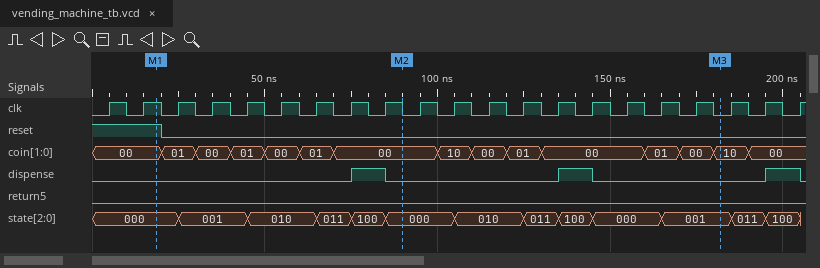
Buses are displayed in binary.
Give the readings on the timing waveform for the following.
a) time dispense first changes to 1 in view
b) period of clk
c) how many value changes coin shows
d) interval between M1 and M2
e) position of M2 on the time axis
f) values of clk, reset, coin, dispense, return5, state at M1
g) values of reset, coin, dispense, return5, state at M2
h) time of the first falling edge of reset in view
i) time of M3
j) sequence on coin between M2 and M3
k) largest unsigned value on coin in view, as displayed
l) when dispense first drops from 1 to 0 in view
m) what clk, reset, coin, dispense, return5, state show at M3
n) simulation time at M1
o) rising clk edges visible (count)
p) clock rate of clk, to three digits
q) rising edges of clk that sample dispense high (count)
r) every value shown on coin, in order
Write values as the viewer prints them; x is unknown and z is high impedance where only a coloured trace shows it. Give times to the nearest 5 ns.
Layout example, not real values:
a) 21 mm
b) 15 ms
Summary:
a) 75 ns
b) 10 ns
c) 14
d) 70 ns
e) 90 ns
f) clk=1, reset=1, coin=00, dispense=0, return5=0, state=000
g) reset=0, coin=00, dispense=0, return5=0, state=000
h) 20 ns
i) 180 ns
j) 00, 10, 00, 01, 00, 01, 00, 10
k) 10
l) 85 ns
m) clk=0, reset=0, coin=10, dispense=0, return5=0, state=001
n) 20 ns
o) 21
p) 100 MHz
q) 3
r) 00, 01, 00, 01, 00, 01, 00, 10, 00, 01, 00, 01, 00, 10, 00
